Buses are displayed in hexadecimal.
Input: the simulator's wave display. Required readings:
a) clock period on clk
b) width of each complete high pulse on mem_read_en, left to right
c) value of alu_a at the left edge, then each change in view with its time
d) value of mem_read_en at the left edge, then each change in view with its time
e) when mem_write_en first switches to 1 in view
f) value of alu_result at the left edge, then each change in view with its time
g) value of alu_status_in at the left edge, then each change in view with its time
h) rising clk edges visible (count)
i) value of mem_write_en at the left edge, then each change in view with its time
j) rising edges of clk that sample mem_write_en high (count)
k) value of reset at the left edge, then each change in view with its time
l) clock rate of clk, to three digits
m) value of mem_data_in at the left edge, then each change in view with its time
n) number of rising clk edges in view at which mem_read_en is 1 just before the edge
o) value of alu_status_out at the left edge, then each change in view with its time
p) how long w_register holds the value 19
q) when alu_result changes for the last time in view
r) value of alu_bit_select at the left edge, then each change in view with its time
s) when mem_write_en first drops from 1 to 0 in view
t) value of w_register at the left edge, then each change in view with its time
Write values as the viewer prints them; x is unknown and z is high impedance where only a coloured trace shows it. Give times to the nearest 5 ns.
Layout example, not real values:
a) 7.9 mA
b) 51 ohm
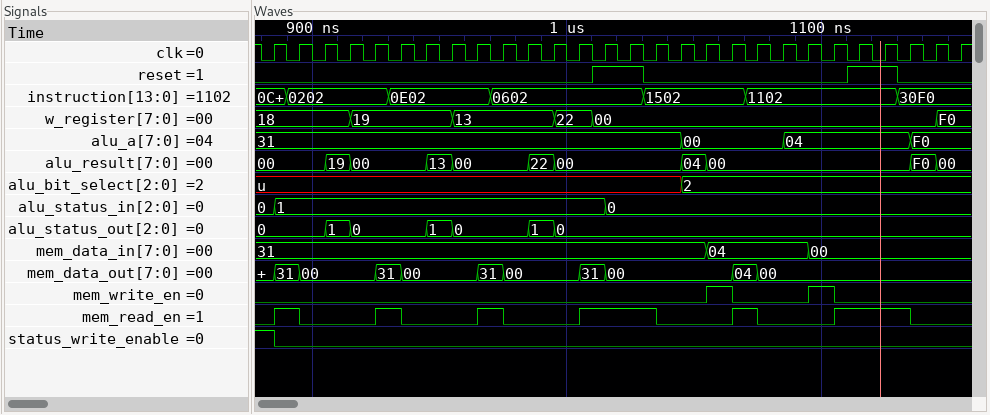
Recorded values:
a) 10 ns
b) 10 ns, 10 ns, 10 ns, 30 ns, 10 ns, 30 ns
c) 31, 00 at 1045 ns, 04 at 1085 ns, F0 at 1135 ns
d) 0, 1 at 885 ns, 0 at 895 ns, 1 at 925 ns, 0 at 935 ns, 1 at 965 ns, 0 at 975 ns, 1 at 1005 ns, 0 at 1035 ns, 1 at 1065 ns, 0 at 1075 ns, 1 at 1105 ns, 0 at 1135 ns
e) 1055 ns
f) 00, 19 at 905 ns, 00 at 915 ns, 13 at 945 ns, 00 at 955 ns, 22 at 985 ns, 00 at 995 ns, 04 at 1045 ns, 00 at 1055 ns, F0 at 1135 ns, 00 at 1145 ns
g) 0, 1 at 885 ns, 0 at 1015 ns
h) 28
i) 0, 1 at 1055 ns, 0 at 1065 ns, 1 at 1095 ns, 0 at 1105 ns
j) 2
k) 0, 1 at 1010 ns, 0 at 1030 ns, 1 at 1110 ns, 0 at 1130 ns
l) 100 MHz
m) 31, 04 at 1055 ns, 00 at 1095 ns
n) 10
o) 0, 1 at 905 ns, 0 at 915 ns, 1 at 945 ns, 0 at 955 ns, 1 at 985 ns, 0 at 995 ns
p) 40 ns
q) 1145 ns
r) u, 2 at 1045 ns
s) 1065 ns
t) 18, 19 at 915 ns, 13 at 955 ns, 22 at 995 ns, 00 at 1010 ns, F0 at 1145 ns
